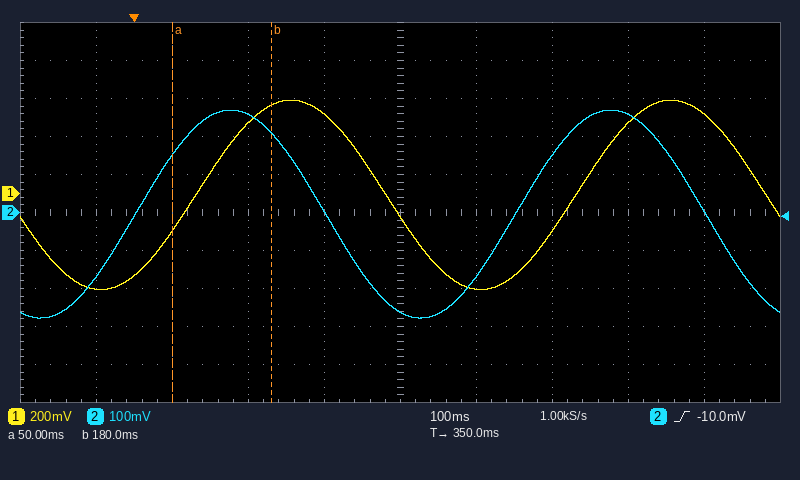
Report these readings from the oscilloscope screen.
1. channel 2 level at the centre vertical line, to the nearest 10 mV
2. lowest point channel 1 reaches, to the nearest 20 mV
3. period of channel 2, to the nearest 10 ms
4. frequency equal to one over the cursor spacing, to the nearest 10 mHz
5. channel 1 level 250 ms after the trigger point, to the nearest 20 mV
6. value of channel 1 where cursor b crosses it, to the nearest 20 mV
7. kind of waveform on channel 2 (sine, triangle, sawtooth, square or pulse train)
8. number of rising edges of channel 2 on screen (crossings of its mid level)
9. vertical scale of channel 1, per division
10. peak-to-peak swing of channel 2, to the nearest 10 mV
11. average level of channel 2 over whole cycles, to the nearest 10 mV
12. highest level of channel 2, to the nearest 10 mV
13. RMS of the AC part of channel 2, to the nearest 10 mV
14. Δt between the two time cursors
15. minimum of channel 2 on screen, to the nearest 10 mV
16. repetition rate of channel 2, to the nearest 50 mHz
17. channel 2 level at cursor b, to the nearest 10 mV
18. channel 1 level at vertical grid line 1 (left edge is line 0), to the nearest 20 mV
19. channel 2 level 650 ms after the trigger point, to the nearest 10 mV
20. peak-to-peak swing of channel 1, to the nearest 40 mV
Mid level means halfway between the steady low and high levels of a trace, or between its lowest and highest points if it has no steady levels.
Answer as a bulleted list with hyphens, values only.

- -260 mV
- -500 mV
- 500 ms
- 7.69 Hz
- 420 mV
- 460 mV
- sine
- 2
- 200 mV
- 550 mV
- 0 mV
- 270 mV
- 190 mV
- 130 ms
- -280 mV
- 2.00 Hz
- 210 mV
- -500 mV
- 260 mV
- 1.00 V
